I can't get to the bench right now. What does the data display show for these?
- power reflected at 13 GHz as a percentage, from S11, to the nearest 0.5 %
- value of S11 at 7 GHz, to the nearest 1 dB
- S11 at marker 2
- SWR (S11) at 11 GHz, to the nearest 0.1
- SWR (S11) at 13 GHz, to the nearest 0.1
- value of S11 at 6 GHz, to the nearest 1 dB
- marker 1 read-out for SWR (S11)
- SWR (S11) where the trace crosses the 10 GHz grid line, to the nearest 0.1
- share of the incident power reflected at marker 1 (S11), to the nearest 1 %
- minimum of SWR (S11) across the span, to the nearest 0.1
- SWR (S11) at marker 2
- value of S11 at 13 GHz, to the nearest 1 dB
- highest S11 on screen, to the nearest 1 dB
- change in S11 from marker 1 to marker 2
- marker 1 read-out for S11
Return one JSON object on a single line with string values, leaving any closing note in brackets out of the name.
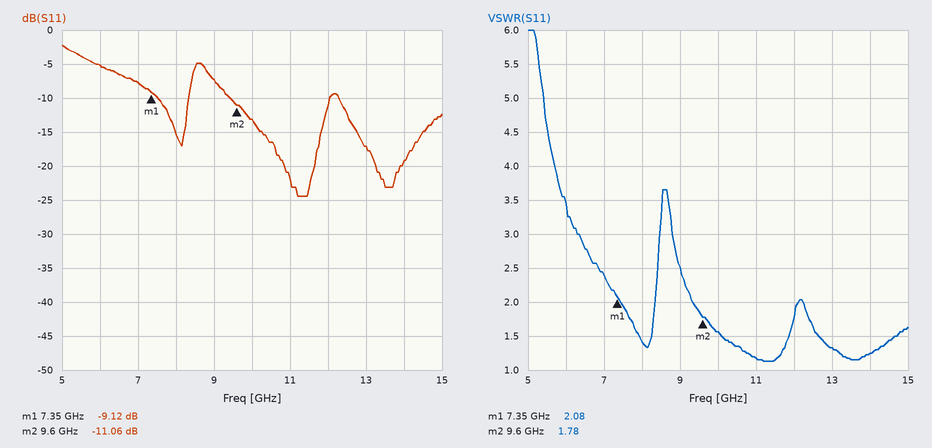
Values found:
{"power reflected at 13 GHz as a percentage, from S11, to the nearest 0.5 %": "2.0 %", "value of S11 at 7 GHz, to the nearest 1 dB": "-8 dB", "S11 at marker 2": "-11.06 dB", "SWR (S11) at 11 GHz, to the nearest 0.1": "1.2", "SWR (S11) at 13 GHz, to the nearest 0.1": "1.3", "value of S11 at 6 GHz, to the nearest 1 dB": "-5 dB", "marker 1 read-out for SWR": "2.08", "SWR (S11) where the trace crosses the 10 GHz grid line, to the nearest 0.1": "1.6", "share of the incident power reflected at marker 1 (S11), to the nearest 1 %": "12 %", "minimum of SWR (S11) across the span, to the nearest 0.1": "1.1", "SWR (S11) at marker 2": "1.78", "value of S11 at 13 GHz, to the nearest 1 dB": "-17 dB", "highest S11 on screen, to the nearest 1 dB": "-2 dB", "change in S11 from marker 1 to marker 2": "-1.94 dB", "marker 1 read-out for S11": "-9.12 dB"}
